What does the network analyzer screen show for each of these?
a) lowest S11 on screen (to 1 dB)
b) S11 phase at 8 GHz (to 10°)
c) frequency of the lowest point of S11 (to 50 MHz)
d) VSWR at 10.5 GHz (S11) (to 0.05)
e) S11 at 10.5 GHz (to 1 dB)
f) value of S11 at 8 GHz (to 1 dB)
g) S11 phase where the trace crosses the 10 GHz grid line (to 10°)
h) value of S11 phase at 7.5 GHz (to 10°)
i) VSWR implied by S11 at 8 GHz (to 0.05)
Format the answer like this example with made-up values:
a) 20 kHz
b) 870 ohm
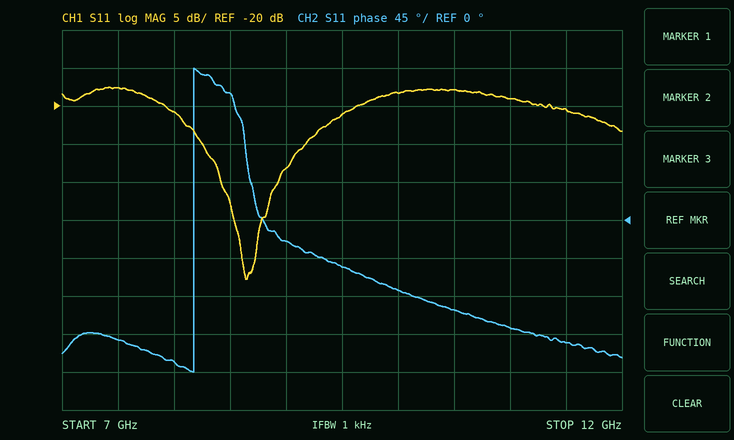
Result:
a) -43 dB
b) -170°
c) 8.65 GHz
d) 1.30
e) -18 dB
f) -21 dB
g) -80°
h) -140°
i) 1.20
